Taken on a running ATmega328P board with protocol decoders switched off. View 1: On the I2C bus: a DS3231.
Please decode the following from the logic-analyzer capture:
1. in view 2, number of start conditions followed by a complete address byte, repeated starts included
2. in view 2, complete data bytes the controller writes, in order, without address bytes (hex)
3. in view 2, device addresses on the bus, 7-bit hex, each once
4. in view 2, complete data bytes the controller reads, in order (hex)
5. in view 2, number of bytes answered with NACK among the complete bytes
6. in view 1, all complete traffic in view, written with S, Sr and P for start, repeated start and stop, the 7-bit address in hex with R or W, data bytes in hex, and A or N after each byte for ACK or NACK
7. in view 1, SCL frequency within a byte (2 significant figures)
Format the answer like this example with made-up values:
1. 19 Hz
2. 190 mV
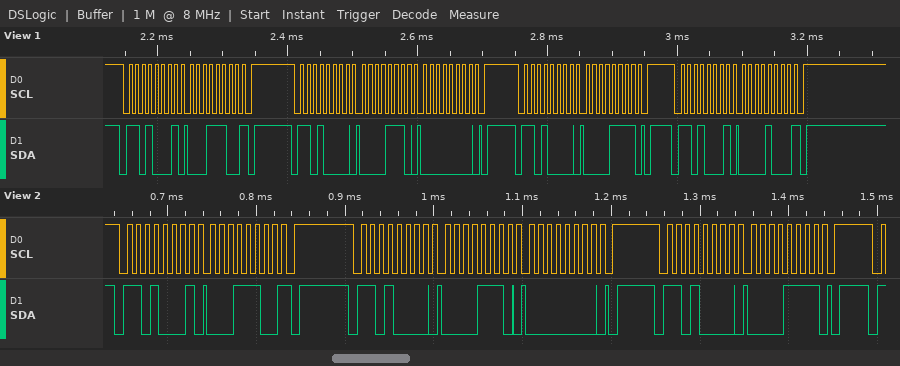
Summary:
1. 3
2. 0E 00 0F
3. 0x68
4. 1C
5. 1
6. S 68R A 1C N P S 68W A 0E A 00 A P S 68W A 0F A P S 68R A 08 N P
7. 100 kHz
